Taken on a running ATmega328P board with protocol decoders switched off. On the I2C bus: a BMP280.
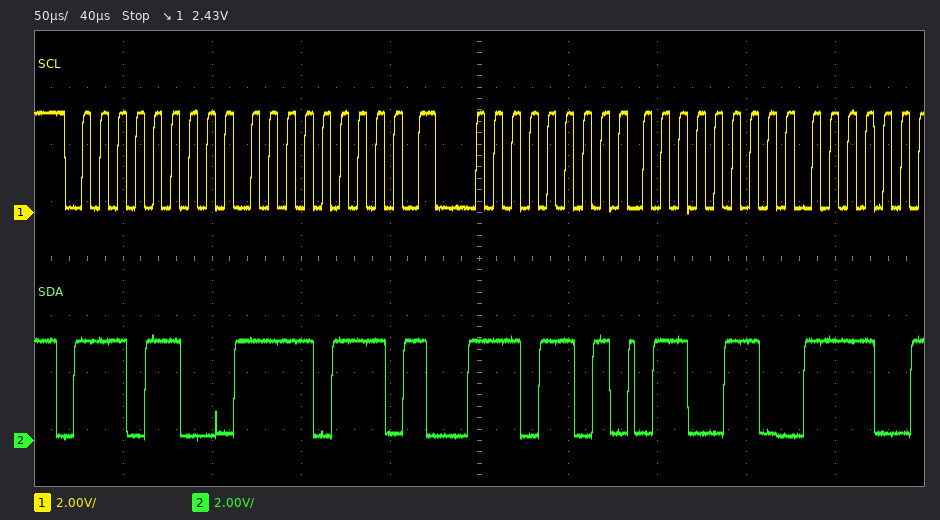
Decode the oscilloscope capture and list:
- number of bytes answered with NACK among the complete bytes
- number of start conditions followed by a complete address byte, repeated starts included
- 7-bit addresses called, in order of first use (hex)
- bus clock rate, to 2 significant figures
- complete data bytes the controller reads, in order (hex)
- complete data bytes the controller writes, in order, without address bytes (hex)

0
2
0x76
100 kHz
66
F7
